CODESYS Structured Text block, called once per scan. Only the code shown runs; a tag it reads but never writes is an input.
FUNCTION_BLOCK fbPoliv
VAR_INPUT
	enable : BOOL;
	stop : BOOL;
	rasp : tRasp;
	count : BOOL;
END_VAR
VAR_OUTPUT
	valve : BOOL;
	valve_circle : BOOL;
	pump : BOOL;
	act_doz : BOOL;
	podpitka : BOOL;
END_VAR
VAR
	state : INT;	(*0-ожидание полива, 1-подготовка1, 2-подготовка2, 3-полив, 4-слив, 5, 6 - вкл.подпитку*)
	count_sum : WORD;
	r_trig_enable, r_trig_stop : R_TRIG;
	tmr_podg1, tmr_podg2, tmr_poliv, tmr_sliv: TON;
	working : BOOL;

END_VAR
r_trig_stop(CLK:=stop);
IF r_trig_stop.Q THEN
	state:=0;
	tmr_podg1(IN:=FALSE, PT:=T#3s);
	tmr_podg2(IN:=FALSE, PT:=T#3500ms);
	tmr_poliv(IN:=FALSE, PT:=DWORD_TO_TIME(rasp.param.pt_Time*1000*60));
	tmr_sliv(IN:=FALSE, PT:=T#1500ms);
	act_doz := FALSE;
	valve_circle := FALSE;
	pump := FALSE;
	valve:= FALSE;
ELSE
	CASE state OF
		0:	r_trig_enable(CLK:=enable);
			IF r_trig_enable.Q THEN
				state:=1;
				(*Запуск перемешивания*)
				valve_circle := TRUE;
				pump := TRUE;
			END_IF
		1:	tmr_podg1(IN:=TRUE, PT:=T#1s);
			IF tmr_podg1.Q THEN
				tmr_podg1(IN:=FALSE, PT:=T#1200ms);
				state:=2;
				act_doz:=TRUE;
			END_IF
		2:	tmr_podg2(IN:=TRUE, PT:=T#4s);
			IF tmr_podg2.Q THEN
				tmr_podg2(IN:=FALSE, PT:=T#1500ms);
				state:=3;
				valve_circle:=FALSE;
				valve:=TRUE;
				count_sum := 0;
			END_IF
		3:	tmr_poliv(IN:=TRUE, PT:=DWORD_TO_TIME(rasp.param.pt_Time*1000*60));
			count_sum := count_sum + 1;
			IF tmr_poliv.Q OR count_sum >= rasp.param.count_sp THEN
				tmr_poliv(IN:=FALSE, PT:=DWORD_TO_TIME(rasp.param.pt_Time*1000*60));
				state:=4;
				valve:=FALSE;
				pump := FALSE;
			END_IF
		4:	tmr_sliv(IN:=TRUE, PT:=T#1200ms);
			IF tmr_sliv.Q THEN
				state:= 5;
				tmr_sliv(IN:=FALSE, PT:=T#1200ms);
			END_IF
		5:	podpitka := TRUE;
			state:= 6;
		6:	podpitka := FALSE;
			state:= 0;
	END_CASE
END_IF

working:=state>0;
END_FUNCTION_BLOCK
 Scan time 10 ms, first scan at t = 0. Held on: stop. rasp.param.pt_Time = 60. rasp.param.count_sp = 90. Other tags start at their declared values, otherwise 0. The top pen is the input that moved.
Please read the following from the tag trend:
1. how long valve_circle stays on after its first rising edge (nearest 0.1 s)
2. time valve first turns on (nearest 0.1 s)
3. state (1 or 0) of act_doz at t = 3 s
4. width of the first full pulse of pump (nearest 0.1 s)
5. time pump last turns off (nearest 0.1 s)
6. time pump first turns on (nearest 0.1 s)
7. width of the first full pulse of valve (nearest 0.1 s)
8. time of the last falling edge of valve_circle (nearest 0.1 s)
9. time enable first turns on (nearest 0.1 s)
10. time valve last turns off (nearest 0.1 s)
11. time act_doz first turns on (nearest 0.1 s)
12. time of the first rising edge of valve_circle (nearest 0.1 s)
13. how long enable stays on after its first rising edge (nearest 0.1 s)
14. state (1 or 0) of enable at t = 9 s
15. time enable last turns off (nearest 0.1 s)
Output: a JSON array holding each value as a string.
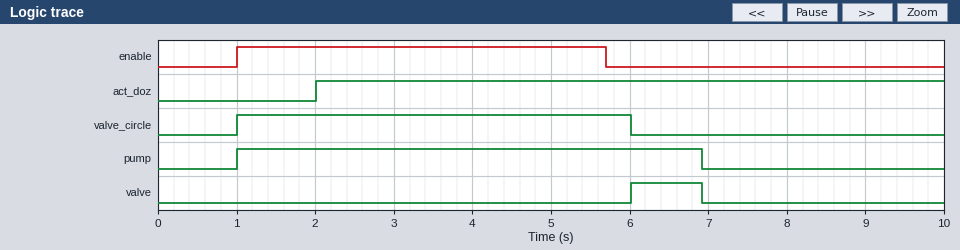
["5.0 s", "6.0 s", "1", "5.9 s", "6.9 s", "1.0 s", "0.9 s", "6.0 s", "1.0 s", "6.9 s", "2.0 s", "1.0 s", "4.7 s", "0", "5.7 s"]
